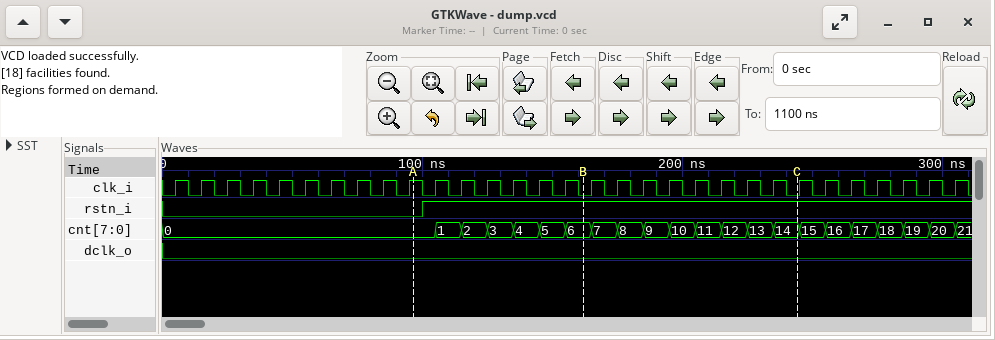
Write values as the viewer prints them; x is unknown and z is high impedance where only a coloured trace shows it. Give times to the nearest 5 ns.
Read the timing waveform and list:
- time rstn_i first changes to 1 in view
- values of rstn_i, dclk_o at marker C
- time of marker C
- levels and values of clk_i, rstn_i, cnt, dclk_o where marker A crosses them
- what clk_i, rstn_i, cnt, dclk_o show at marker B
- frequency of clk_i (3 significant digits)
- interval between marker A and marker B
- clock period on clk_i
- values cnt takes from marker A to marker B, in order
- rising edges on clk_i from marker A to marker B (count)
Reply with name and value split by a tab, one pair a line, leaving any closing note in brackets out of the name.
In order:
time rstn_i first changes to 1 in view	100 ns
values of rstn_i, dclk_o at marker C	rstn_i=1, dclk_o=0
time of marker C	245 ns
levels and values of clk_i, rstn_i, cnt, dclk_o where marker A crosses them	clk_i=1, rstn_i=0, cnt=0, dclk_o=0
what clk_i, rstn_i, cnt, dclk_o show at marker B	clk_i=0, rstn_i=1, cnt=6, dclk_o=0
frequency of clk_i	100 MHz
interval between marker A and marker B	65 ns
clock period on clk_i	10 ns
values cnt takes from marker A to marker B, in order	0, 1, 2, 3, 4, 5, 6
rising edges on clk_i from marker A to marker B	6
